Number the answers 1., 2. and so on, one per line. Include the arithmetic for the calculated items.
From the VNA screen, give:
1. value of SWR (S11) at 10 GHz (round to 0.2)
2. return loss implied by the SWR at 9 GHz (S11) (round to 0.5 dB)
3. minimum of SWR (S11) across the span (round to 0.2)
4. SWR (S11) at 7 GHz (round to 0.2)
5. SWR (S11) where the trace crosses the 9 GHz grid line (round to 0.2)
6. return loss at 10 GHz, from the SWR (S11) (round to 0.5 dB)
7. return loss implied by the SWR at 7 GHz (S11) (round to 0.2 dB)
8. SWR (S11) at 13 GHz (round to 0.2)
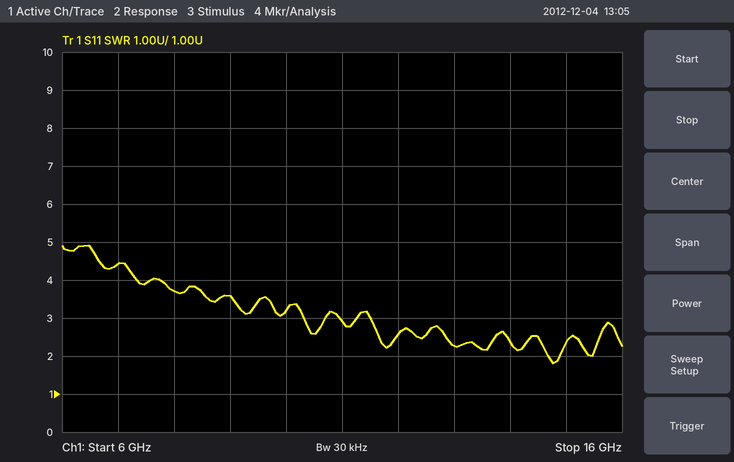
1. 3.2
2. −20 log10((3.6 − 1)/(3.6 + 1)) ≈ 5.0 dB
3. 1.8
4. 4.4
5. 3.6
6. −20 log10((3.2 − 1)/(3.2 + 1)) ≈ 5.62 dB, so 5.5 dB to the nearest 0.5 dB
7. −20 log10((4.4 − 1)/(4.4 + 1)) ≈ 4.0 dB
8. 2.2
